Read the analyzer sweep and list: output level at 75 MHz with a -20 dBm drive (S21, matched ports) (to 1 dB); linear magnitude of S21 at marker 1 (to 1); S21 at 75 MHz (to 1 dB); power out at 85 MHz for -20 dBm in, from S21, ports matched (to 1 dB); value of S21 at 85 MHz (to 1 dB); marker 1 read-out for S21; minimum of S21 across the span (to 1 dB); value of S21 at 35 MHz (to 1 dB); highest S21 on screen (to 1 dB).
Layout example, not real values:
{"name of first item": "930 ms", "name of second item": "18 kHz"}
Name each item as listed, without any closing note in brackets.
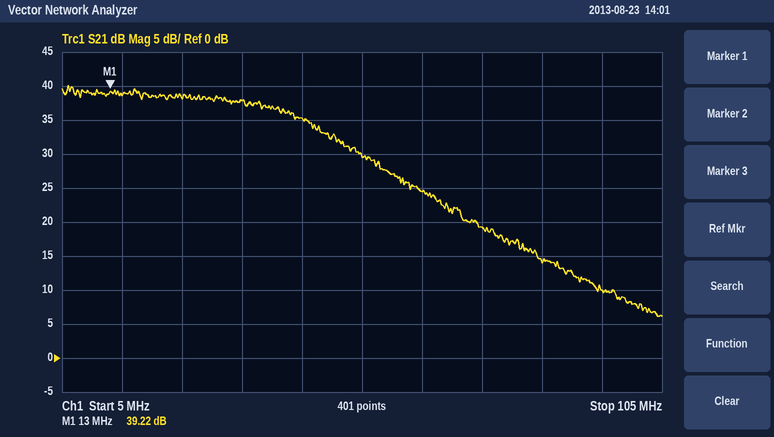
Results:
{"output level at 75 MHz with a -20 dBm drive (S21, matched ports)": "-1 dBm", "linear magnitude of S21 at marker 1": "91", "S21 at 75 MHz": "19 dB", "power out at 85 MHz for -20 dBm in, from S21, ports matched": "-6 dBm", "value of S21 at 85 MHz": "14 dB", "marker 1 read-out for S21": "39.22 dB", "minimum of S21 across the span": "6 dB", "value of S21 at 35 MHz": "38 dB", "highest S21 on screen": "40 dB"}
